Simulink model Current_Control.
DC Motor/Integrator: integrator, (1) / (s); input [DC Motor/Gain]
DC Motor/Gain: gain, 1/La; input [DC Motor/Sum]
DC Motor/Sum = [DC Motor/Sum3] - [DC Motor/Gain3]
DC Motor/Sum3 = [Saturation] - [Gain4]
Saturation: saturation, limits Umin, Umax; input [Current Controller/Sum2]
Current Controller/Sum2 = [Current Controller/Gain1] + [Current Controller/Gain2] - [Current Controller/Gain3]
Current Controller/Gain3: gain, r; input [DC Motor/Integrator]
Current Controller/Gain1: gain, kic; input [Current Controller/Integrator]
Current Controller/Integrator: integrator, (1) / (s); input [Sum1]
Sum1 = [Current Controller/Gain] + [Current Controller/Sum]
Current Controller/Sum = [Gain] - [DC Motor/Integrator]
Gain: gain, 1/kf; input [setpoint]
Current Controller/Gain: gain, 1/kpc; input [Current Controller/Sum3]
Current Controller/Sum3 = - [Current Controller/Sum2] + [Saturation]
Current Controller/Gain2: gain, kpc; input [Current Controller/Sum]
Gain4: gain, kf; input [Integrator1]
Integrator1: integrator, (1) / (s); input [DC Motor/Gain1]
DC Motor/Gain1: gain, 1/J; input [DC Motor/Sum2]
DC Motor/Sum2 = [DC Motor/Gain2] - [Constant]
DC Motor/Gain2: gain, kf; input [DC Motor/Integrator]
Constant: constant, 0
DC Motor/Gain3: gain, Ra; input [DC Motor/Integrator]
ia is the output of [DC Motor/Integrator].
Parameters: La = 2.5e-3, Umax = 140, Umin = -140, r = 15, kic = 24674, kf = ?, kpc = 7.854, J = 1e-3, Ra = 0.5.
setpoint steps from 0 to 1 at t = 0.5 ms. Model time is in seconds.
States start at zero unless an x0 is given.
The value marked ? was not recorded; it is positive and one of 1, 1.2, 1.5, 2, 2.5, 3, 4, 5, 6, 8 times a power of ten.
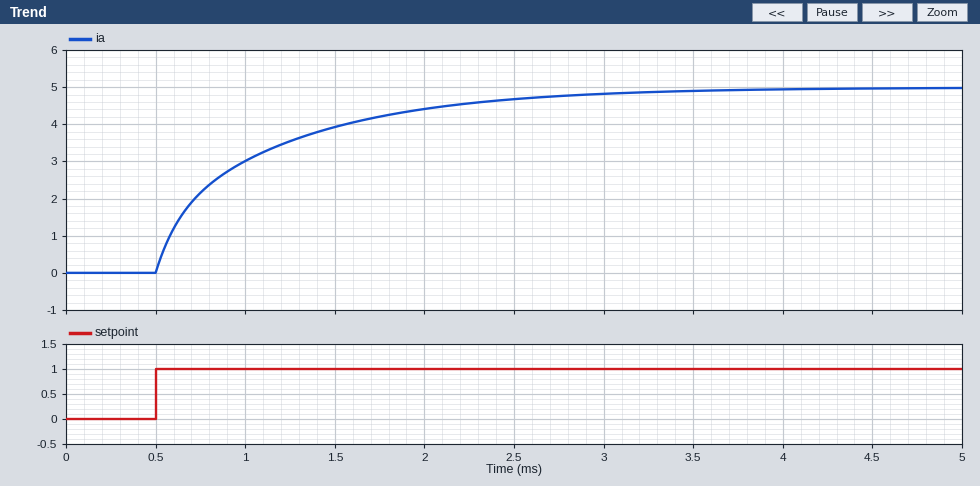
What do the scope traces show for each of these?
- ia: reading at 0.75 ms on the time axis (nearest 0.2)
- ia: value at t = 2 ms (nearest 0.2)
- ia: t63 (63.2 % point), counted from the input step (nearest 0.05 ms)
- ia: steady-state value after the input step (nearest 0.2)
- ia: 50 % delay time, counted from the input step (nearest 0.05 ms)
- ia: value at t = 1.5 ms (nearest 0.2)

2.2
4.4
0.55 ms
5.0
0.35 ms
4.0
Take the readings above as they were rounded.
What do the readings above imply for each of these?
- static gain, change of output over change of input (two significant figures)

5.0
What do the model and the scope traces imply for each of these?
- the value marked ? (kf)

0.2
